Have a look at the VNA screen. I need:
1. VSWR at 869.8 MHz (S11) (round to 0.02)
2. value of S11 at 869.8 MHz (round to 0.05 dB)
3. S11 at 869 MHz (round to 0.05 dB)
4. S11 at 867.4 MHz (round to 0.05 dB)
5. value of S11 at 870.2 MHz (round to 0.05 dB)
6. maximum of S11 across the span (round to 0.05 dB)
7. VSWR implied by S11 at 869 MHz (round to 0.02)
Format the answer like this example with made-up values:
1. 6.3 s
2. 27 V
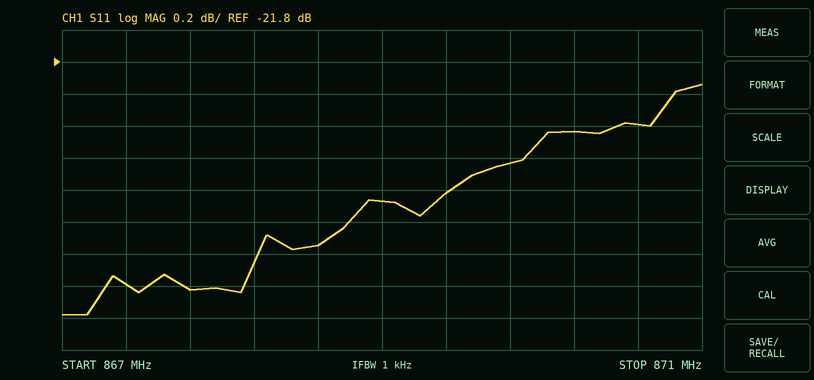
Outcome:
1. 1.16
2. -22.45 dB
3. -22.65 dB
4. -23.20 dB
5. -22.25 dB
6. -21.95 dB
7. 1.16
